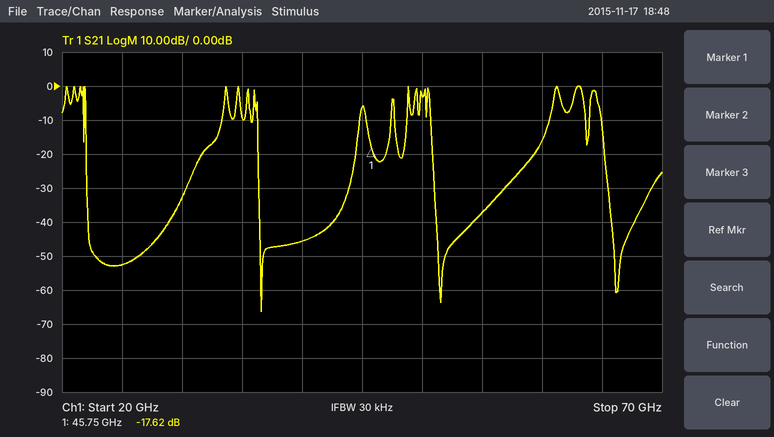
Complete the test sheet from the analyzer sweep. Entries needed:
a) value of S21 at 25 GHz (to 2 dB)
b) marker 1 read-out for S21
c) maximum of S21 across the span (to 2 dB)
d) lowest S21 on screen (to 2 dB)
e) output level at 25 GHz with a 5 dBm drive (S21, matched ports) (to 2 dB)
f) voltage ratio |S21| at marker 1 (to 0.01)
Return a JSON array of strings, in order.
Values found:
["-52 dB", "-17.62 dB", "0 dB", "-66 dB", "-48 dBm", "0.13"]
